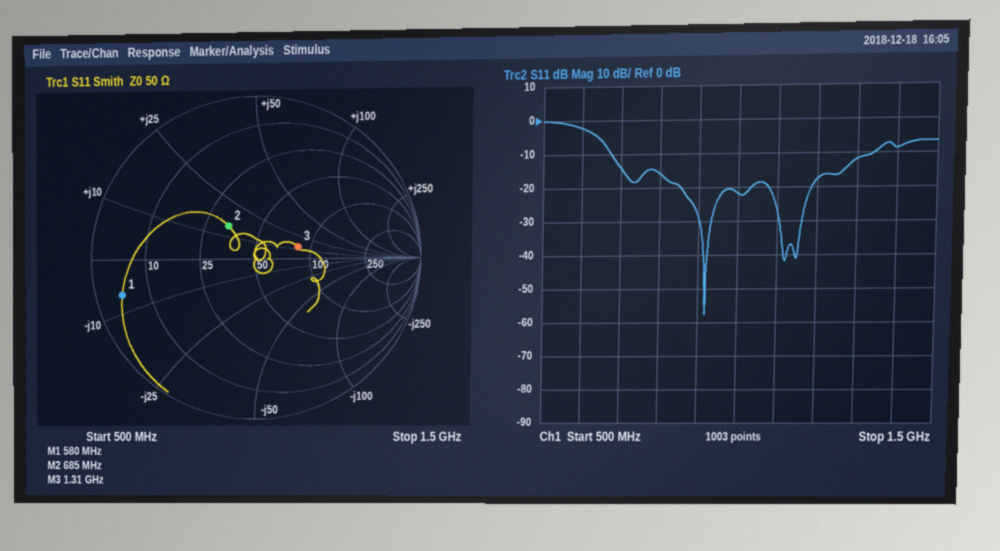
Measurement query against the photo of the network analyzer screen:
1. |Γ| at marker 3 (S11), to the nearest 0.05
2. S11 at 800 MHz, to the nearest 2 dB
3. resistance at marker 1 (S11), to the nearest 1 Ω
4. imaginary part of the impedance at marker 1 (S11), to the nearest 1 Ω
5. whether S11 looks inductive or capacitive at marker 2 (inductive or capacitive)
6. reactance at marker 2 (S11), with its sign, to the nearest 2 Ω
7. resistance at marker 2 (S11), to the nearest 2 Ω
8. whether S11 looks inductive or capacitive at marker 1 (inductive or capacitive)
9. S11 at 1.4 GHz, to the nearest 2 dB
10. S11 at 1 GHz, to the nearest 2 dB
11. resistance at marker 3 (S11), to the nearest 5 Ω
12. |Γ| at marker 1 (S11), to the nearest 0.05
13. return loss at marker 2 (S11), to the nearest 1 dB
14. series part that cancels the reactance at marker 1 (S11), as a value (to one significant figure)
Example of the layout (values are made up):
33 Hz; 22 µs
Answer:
0.25; -16 dB; 4 Ω; -7 Ω; inductive; +14 Ω; 34 Ω; capacitive; -8 dB; -22 dB; 85 Ω; 0.85; 12 dB; 2 nH
